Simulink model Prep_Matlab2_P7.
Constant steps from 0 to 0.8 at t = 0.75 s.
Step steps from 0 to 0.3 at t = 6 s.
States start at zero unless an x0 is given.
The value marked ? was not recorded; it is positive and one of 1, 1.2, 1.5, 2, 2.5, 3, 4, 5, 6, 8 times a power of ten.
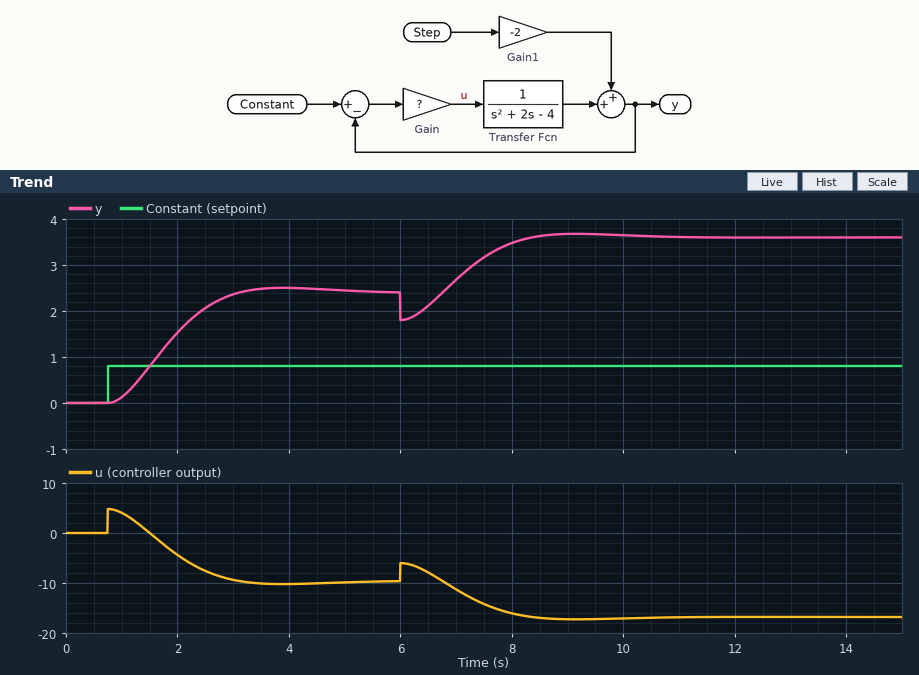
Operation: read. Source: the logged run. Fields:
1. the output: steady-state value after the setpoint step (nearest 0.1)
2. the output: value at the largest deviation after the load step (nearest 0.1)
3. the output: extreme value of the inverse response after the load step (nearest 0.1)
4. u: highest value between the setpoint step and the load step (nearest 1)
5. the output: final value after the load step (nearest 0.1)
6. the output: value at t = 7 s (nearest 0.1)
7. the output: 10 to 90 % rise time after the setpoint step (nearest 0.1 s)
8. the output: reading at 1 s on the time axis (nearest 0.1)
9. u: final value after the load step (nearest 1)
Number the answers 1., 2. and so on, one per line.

1. 2.4
2. 3.7
3. 1.8
4. 5
5. 3.6
6. 2.7
7. 1.5 s
8. 0.1
9. -17
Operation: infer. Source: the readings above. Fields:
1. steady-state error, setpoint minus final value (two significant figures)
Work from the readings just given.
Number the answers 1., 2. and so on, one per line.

1. -1.6
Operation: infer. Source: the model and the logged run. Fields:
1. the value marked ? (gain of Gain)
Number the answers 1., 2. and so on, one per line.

1. 6
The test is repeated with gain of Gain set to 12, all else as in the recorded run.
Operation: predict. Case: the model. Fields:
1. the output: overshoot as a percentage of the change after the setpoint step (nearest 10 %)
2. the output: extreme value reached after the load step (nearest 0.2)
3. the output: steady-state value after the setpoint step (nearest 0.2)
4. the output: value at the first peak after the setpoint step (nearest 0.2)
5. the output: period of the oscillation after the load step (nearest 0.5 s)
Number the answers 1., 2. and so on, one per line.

1. 30 %
2. 1.8
3. 1.2
4. 1.6
5. 2.5 s
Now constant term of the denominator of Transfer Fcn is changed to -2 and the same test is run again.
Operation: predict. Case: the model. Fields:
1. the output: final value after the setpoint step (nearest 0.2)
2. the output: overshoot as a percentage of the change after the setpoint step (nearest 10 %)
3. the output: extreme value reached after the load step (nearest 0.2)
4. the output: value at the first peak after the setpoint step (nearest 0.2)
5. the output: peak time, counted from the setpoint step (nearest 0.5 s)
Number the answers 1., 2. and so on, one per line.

1. 1.2
2. 20 %
3. 1.6
4. 1.4
5. 2.0 s
